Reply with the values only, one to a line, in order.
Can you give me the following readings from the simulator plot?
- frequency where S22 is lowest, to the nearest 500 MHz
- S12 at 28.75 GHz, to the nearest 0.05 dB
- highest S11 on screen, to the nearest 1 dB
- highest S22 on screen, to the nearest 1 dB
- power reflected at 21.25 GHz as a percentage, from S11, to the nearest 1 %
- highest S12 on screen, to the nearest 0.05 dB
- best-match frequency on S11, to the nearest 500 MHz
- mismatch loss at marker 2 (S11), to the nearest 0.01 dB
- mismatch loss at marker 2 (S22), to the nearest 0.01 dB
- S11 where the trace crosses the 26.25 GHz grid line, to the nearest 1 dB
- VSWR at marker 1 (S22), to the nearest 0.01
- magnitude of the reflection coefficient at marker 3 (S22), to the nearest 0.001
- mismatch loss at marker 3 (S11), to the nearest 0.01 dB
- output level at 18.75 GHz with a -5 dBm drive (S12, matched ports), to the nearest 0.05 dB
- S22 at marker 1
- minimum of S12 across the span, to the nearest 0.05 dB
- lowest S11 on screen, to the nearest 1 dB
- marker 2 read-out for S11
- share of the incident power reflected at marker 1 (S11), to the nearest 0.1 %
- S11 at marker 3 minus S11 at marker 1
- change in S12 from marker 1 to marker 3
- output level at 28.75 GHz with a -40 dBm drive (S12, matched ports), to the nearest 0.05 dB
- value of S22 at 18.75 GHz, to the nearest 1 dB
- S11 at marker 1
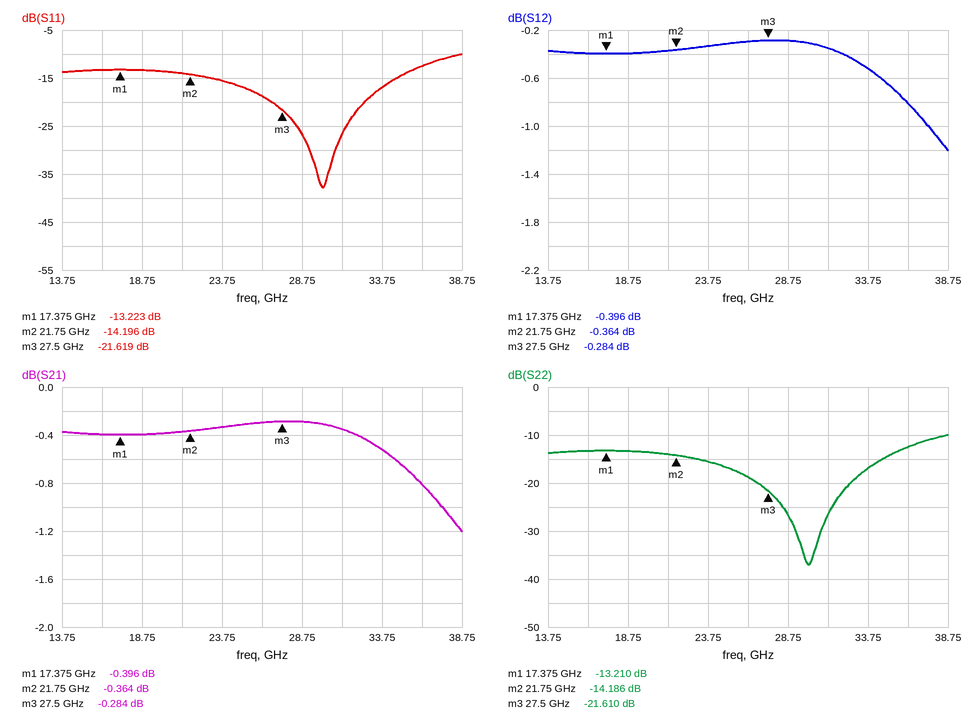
30.0 GHz
-0.30 dB
-10 dB
-10 dB
4 %
-0.30 dB
30.0 GHz
0.17 dB
0.17 dB
-19 dB
1.56
0.083
0.03 dB
-5.40 dBm
-13.210 dB
-1.20 dB
-38 dB
-14.196 dB
4.8 %
-8.396 dB
0.112 dB
-40.30 dBm
-13 dB
-13.223 dB
